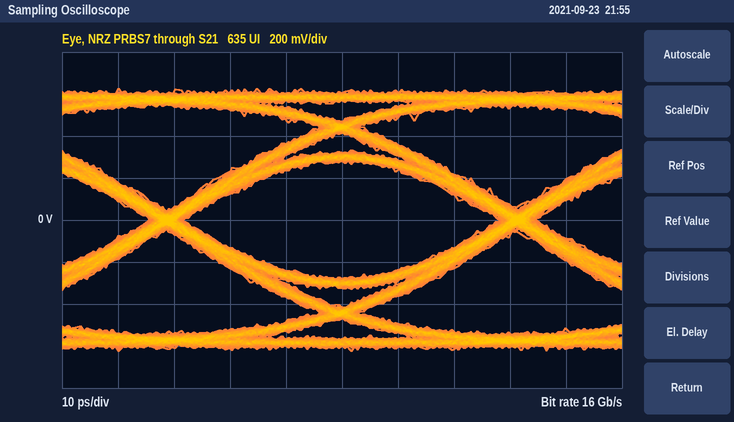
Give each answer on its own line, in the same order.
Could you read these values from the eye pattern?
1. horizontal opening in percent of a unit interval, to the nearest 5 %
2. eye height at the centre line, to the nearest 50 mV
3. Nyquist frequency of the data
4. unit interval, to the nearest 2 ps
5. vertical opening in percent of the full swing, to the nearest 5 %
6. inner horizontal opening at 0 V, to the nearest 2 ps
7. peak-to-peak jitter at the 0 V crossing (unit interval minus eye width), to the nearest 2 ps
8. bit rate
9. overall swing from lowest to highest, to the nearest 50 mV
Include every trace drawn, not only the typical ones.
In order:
90 %
550 mV
8 GHz
62 ps
45 %
56 ps
6 ps
16 Gb/s
1.25 V
